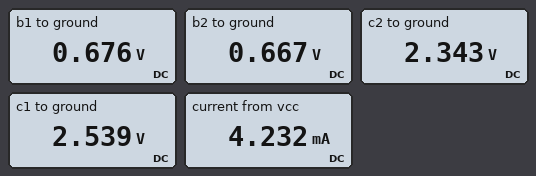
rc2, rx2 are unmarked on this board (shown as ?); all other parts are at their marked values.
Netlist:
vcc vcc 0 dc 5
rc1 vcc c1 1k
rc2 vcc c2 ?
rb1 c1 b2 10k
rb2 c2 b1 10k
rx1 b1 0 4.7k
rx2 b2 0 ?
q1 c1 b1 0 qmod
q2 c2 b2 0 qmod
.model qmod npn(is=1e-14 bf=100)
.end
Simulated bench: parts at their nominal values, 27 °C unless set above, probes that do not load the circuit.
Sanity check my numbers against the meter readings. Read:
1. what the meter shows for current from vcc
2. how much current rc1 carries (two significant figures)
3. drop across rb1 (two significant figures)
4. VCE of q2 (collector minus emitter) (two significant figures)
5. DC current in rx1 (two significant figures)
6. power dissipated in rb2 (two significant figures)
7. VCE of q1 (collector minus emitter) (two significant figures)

4.232 mA
2.5 mA
1.9 V
2.3 V
140 µA
280 µW
2.5 V
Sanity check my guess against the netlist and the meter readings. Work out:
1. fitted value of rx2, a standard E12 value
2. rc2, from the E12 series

3.9 kΩ
1.5 kΩ
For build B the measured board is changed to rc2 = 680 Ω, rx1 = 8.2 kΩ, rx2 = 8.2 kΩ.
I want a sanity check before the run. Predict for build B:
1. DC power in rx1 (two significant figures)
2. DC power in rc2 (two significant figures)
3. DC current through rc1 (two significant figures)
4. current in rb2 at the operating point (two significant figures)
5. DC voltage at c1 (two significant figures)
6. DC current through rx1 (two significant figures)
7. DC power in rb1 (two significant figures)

57 µW
15 mW
3.0 mA
110 µA
2.0 V
83 µA
170 µW
